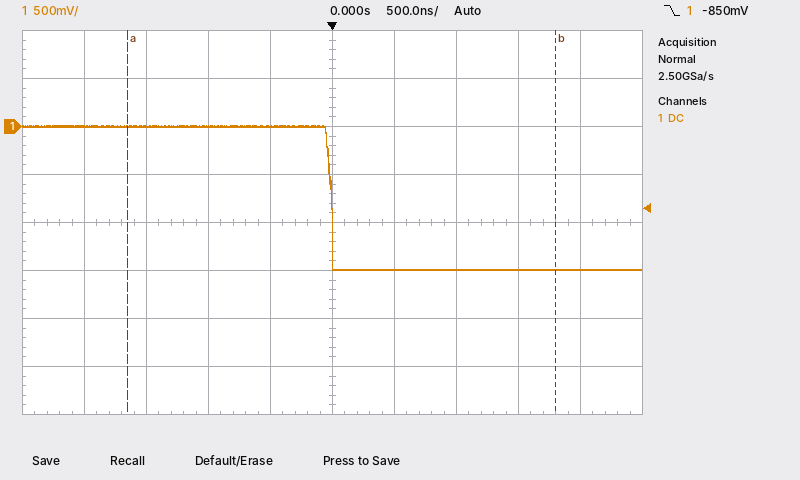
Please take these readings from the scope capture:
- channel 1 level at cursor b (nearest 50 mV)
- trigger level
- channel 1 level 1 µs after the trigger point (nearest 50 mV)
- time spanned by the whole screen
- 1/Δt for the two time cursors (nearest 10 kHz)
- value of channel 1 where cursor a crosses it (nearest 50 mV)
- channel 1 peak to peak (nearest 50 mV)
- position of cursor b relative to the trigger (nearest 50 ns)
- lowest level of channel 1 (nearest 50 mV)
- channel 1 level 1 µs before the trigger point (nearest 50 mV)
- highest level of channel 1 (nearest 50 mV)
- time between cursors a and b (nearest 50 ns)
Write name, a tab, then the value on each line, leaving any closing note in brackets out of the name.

channel 1 level at cursor b	-1.50 V
trigger level	-850 mV
channel 1 level 1 µs after the trigger point	-1.50 V
time spanned by the whole screen	5 µs
1/Δt for the two time cursors	290 kHz
value of channel 1 where cursor a crosses it	0 mV
channel 1 peak to peak	1.50 V
position of cursor b relative to the trigger	+1.80 µs
lowest level of channel 1	-1.50 V
channel 1 level 1 µs before the trigger point	0 mV
highest level of channel 1	0 mV
time between cursors a and b	3.45 µs
